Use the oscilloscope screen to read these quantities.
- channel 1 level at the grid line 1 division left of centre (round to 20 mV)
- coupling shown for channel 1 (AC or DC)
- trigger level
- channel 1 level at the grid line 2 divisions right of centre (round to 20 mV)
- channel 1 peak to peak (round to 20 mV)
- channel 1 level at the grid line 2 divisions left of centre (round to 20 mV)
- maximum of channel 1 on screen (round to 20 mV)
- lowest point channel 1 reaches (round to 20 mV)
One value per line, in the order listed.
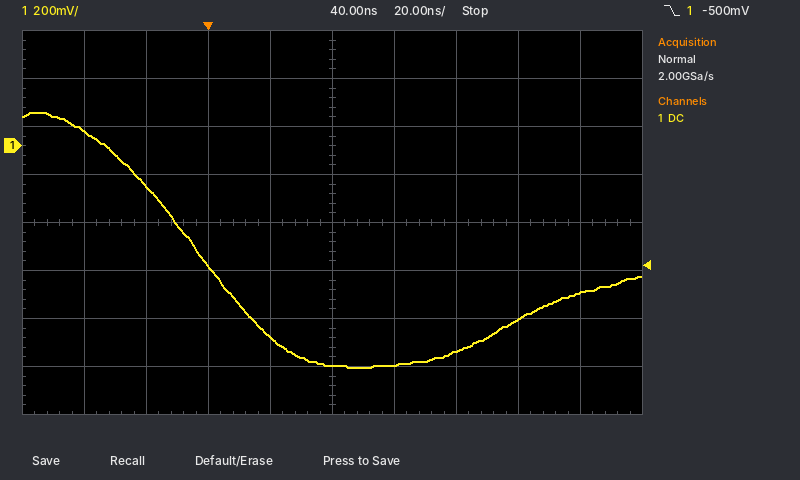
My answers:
-800 mV
DC
-500 mV
-860 mV
1.06 V
-500 mV
140 mV
-920 mV
